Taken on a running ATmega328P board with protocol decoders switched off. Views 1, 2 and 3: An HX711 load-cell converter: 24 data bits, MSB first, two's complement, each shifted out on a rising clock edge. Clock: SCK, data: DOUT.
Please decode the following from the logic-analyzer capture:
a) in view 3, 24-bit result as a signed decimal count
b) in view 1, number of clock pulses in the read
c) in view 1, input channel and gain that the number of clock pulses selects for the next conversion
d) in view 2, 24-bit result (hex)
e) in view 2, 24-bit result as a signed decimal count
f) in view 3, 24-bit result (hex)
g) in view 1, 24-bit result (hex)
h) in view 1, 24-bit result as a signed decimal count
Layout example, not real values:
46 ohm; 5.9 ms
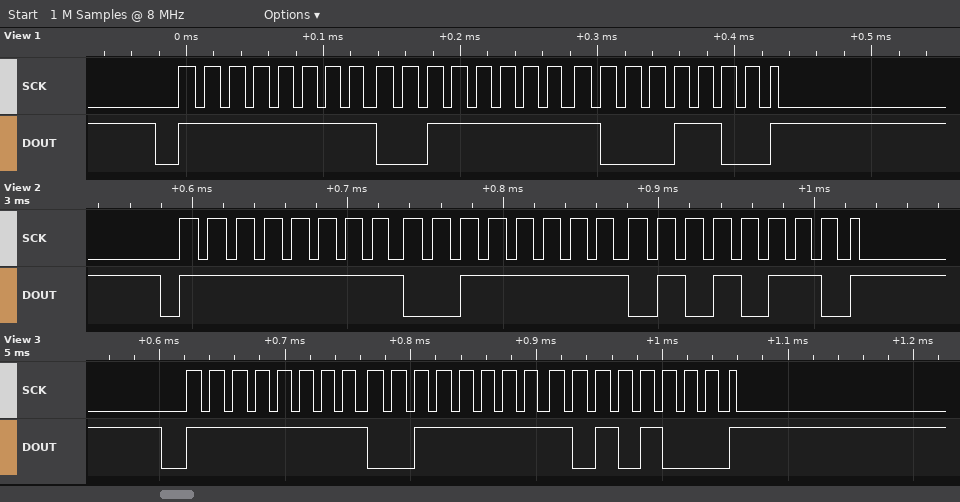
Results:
-49240; 25; channel A, gain 128; 0xFF3F56; -49322; 0xFF3FA8; 0xFF3F8C; -49268
